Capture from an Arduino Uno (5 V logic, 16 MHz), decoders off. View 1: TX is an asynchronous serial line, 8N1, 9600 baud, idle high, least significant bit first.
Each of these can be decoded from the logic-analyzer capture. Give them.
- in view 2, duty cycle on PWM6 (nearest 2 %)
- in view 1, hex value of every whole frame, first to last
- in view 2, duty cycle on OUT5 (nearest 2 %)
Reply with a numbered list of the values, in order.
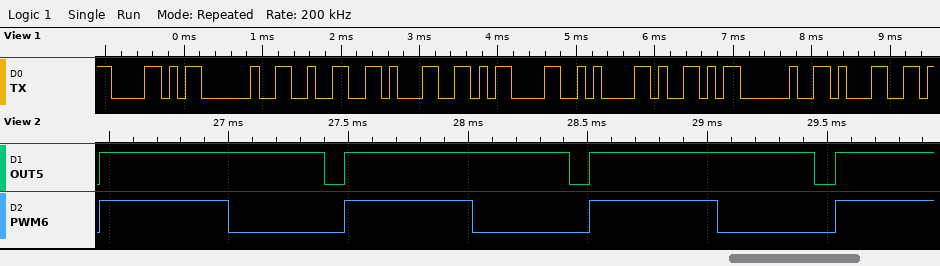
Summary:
1. 52 %
2. 58 20 32 31 0D 0A 59 20 31
3. 92 %
